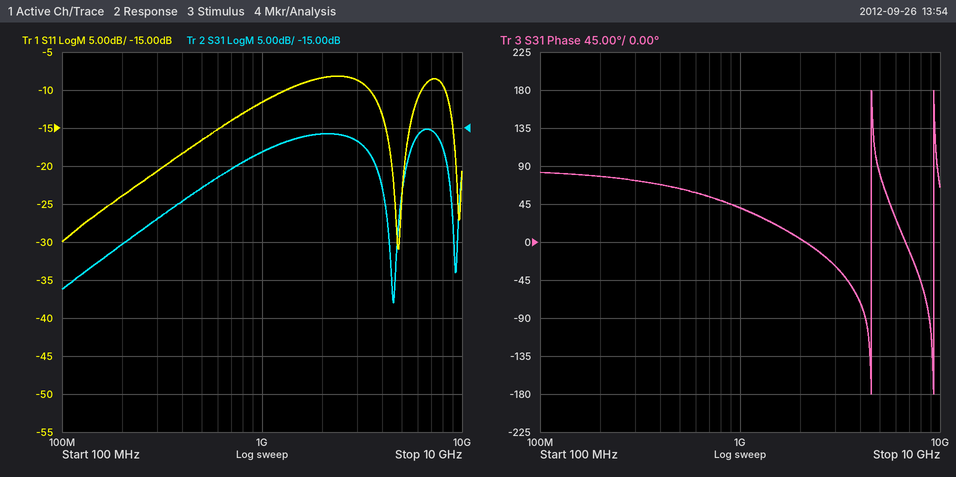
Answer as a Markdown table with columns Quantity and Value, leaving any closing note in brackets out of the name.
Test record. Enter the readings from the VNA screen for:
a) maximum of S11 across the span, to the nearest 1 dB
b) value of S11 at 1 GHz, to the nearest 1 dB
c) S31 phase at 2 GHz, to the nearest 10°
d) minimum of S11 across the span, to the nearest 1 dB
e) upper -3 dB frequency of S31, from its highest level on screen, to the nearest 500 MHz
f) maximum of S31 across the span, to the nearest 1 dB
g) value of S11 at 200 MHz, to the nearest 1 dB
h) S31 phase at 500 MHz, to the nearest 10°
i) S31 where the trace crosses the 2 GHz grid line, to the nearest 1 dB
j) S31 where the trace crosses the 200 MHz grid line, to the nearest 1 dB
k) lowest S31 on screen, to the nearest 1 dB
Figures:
| Quantity | Value |
|---|---|
| maximum of S11 across the span, to the nearest 1 dB | -8 dB |
| value of S11 at 1 GHz, to the nearest 1 dB | -12 dB |
| S31 phase at 2 GHz, to the nearest 10° | 0° |
| minimum of S11 across the span, to the nearest 1 dB | -31 dB |
| upper -3 dB frequency of S31, from its highest level on screen, to the nearest 500 MHz | 8.0 GHz |
| maximum of S31 across the span, to the nearest 1 dB | -15 dB |
| value of S11 at 200 MHz, to the nearest 1 dB | -24 dB |
| S31 phase at 500 MHz, to the nearest 10° | 60° |
| S31 where the trace crosses the 2 GHz grid line, to the nearest 1 dB | -16 dB |
| S31 where the trace crosses the 200 MHz grid line, to the nearest 1 dB | -30 dB |
| lowest S31 on screen, to the nearest 1 dB | -38 dB |
